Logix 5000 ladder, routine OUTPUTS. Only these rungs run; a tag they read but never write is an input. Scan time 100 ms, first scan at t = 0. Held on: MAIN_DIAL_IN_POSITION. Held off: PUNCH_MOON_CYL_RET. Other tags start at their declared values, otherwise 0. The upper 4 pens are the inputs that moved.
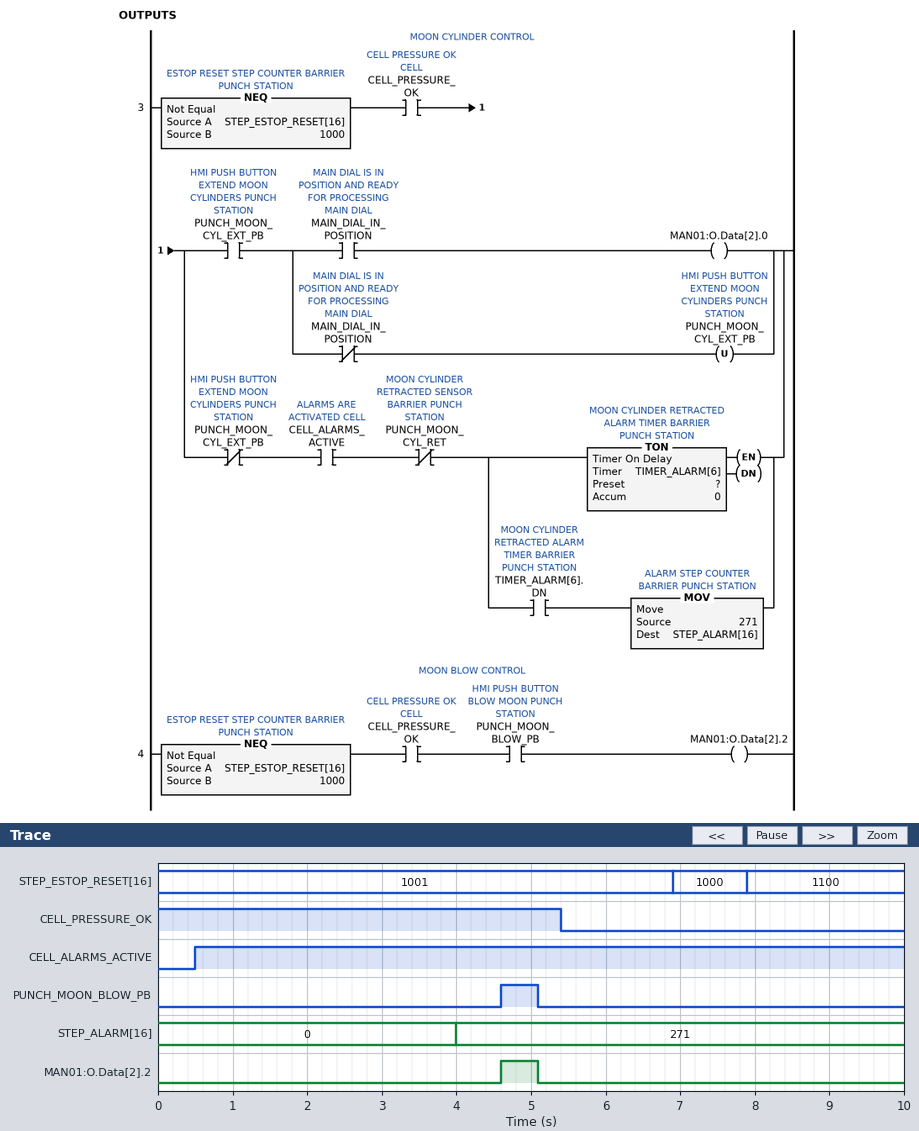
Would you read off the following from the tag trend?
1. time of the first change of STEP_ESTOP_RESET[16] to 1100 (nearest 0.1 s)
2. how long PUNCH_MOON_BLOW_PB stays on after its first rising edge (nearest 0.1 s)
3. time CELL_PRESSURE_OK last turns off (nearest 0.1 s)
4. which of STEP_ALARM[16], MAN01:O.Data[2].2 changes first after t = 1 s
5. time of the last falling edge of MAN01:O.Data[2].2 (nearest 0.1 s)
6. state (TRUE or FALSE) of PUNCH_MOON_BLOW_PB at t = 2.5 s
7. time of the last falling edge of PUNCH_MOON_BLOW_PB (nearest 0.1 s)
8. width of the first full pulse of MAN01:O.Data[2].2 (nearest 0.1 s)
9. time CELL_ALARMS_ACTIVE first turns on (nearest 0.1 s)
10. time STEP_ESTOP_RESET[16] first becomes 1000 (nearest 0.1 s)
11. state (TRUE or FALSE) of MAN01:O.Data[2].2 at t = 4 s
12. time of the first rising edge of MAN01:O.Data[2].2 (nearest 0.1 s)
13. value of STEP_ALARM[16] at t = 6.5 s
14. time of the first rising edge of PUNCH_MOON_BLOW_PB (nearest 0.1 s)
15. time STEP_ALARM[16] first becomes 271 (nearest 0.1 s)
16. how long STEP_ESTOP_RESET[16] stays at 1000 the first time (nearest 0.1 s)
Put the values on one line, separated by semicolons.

7.9 s; 0.5 s; 5.4 s; STEP_ALARM[16]; 5.1 s; FALSE; 5.1 s; 0.5 s; 0.5 s; 6.9 s; FALSE; 4.6 s; 271; 4.6 s; 4.0 s; 1.0 s
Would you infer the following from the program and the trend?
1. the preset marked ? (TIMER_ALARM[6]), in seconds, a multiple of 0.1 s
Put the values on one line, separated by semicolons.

3.5 s
